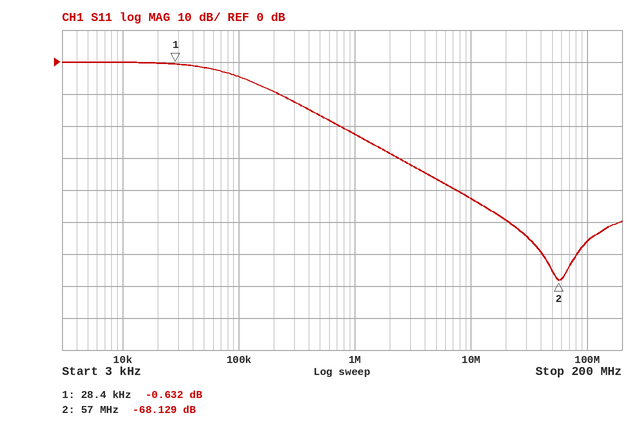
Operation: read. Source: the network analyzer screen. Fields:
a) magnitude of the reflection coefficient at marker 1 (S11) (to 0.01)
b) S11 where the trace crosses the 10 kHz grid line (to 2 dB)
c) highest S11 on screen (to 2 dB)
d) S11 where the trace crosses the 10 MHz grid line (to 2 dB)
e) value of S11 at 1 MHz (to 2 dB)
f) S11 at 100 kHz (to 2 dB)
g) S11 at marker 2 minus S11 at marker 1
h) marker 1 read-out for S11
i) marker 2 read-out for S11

0.93
0 dB
0 dB
-42 dB
-22 dB
-4 dB
-67.497 dB
-0.632 dB
-68.129 dB
